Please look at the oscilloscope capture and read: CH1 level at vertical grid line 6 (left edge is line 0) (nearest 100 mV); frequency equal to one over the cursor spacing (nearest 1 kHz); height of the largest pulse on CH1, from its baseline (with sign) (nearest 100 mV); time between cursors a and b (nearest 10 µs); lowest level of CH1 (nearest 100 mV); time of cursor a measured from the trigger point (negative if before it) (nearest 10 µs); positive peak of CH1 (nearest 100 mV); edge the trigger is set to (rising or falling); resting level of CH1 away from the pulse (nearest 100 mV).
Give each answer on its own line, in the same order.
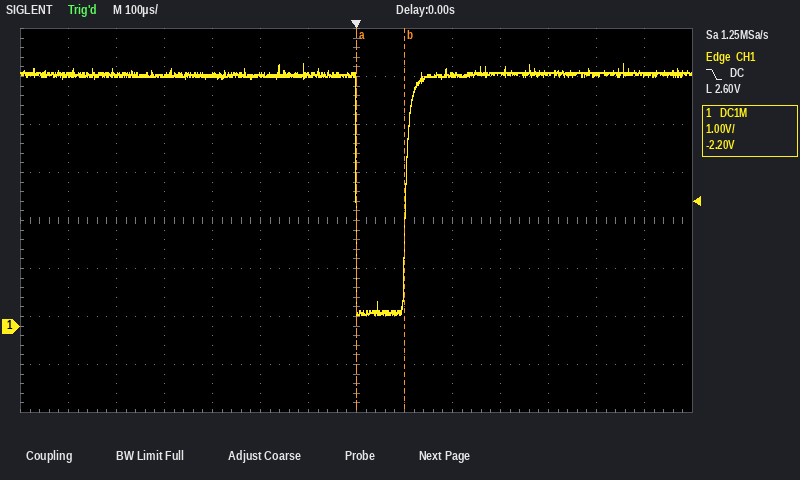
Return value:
5.2 V
10 kHz
-5.0 V
100 µs
200 mV
0 µs
5.5 V
falling
5.2 V
